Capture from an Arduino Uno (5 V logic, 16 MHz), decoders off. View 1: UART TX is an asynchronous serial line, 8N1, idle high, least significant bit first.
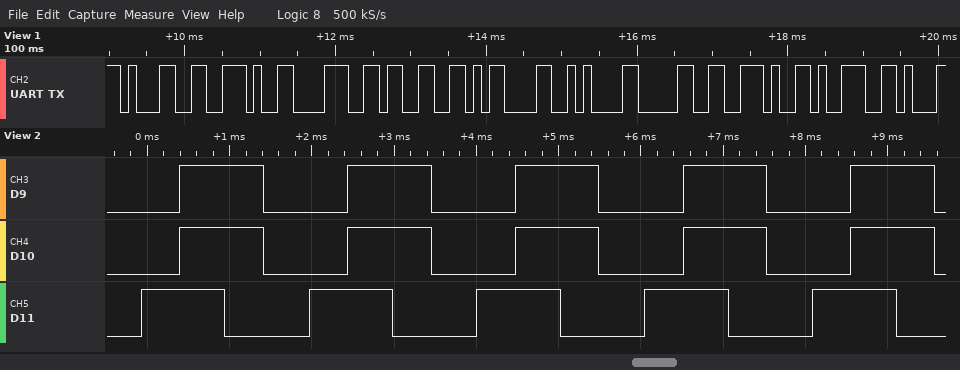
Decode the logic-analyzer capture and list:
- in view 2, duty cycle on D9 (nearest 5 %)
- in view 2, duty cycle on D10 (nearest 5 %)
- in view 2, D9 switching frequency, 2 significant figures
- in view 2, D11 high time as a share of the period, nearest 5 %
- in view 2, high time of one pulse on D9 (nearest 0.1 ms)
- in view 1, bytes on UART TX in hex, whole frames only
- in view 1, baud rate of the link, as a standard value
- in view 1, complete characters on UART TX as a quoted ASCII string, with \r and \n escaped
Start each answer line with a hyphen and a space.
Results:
- 50 %
- 50 %
- 490 Hz
- 50 %
- 1.0 ms
- 31 2E 38 33 0D 0A 30 2E 39
- 9600 baud
- "1.83\r\n0.9"
